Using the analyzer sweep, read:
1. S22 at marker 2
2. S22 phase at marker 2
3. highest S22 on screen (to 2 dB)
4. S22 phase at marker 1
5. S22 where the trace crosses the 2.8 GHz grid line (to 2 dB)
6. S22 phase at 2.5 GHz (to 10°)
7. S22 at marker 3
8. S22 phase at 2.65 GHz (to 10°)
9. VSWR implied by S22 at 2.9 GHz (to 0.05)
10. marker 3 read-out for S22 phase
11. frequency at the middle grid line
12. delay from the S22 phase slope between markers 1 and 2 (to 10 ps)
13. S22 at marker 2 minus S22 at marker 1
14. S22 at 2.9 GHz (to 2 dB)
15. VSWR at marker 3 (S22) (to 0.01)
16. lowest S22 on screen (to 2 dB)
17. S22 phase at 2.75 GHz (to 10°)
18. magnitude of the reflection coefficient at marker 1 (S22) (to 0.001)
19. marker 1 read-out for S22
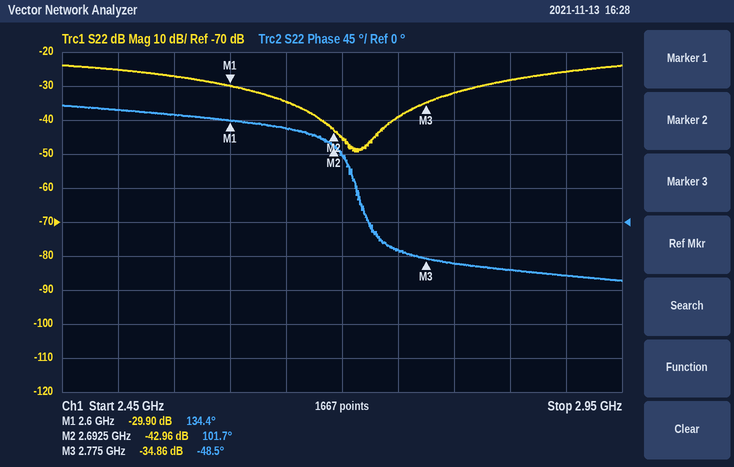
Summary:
-42.96 dB
101.7°
-24 dB
134.4°
-32 dB
150°
-34.86 dB
120°
1.10
-48.5°
2.7 GHz
980 ps
-13.06 dB
-26 dB
1.04
-50 dB
-40°
0.032
-29.90 dB
